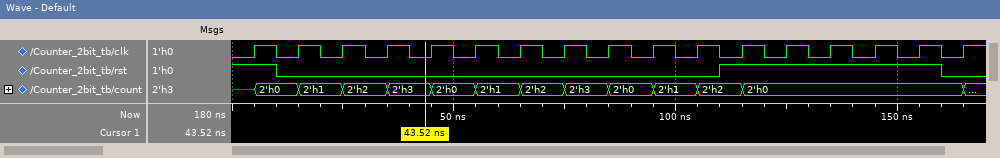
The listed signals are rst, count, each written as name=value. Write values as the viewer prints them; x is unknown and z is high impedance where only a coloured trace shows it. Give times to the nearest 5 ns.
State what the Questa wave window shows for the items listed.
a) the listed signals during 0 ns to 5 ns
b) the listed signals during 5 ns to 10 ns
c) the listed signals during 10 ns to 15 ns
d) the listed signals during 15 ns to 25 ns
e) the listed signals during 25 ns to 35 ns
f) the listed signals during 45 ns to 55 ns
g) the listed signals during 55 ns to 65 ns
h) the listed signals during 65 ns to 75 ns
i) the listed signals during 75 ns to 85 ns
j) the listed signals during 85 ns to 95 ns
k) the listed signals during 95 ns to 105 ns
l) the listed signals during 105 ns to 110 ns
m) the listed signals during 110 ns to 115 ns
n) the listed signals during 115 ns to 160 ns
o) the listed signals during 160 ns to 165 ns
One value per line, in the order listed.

rst=1, count=x
rst=1, count=2'h0
rst=0, count=2'h0
rst=0, count=2'h1
rst=0, count=2'h2
rst=0, count=2'h0
rst=0, count=2'h1
rst=0, count=2'h2
rst=0, count=2'h3
rst=0, count=2'h0
rst=0, count=2'h1
rst=0, count=2'h2
rst=1, count=2'h2
rst=1, count=2'h0
rst=0, count=2'h0
